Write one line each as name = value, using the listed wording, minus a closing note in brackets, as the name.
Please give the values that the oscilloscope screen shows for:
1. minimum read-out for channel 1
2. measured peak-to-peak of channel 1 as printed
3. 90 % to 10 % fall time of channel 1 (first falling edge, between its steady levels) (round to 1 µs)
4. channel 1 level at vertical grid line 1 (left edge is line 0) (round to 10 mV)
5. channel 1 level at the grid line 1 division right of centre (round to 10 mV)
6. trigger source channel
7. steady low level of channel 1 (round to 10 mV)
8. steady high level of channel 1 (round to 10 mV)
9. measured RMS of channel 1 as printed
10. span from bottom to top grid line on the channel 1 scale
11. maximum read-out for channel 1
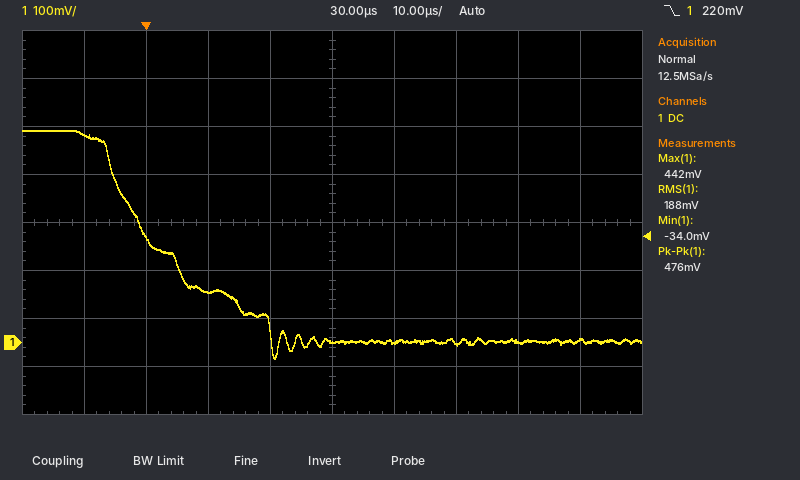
minimum read-out for channel 1 = -34.0 mV
measured peak-to-peak of channel 1 as printed = 476 mV
90 % to 10 % fall time of channel 1 (first falling edge, between its steady levels) = 26 µs
channel 1 level at vertical grid line 1 (left edge is line 0) = 430 mV
channel 1 level at the grid line 1 division right of centre = 0 mV
trigger source channel = channel 1
steady low level of channel 1 = 0 mV
steady high level of channel 1 = 440 mV
measured RMS of channel 1 as printed = 188 mV
span from bottom to top grid line on the channel 1 scale = 800 mV
maximum read-out for channel 1 = 442 mV
